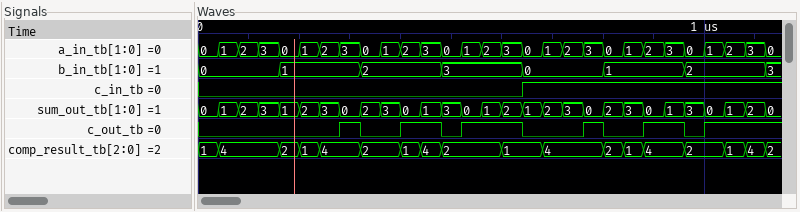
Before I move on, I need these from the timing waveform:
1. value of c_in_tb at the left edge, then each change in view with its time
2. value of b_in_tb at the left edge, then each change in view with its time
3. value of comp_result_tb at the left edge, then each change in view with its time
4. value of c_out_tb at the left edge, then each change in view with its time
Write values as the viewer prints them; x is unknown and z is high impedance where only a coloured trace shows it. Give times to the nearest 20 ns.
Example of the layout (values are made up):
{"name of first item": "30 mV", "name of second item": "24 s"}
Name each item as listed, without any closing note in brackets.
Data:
{"value of c_in_tb at the left edge, then each change in view with its time": "0, 1 at 640 ns", "value of b_in_tb at the left edge, then each change in view with its time": "0, 1 at 160 ns, 2 at 320 ns, 3 at 480 ns, 0 at 640 ns, 1 at 800 ns, 2 at 960 ns, 3 at 1120 ns", "value of comp_result_tb at the left edge, then each change in view with its time": "1, 4 at 40 ns, 2 at 160 ns, 1 at 200 ns, 4 at 240 ns, 2 at 320 ns, 1 at 400 ns, 4 at 440 ns, 2 at 480 ns, 1 at 600 ns, 4 at 680 ns, 2 at 800 ns, 1 at 840 ns, 4 at 880 ns, 2 at 960 ns, 1 at 1040 ns, 4 at 1080 ns, 2 at 1120 ns", "value of c_out_tb at the left edge, then each change in view with its time": "0, 1 at 280 ns, 0 at 320 ns, 1 at 400 ns, 0 at 480 ns, 1 at 520 ns, 0 at 640 ns, 1 at 760 ns, 0 at 800 ns, 1 at 880 ns, 0 at 960 ns, 1 at 1000 ns"}
